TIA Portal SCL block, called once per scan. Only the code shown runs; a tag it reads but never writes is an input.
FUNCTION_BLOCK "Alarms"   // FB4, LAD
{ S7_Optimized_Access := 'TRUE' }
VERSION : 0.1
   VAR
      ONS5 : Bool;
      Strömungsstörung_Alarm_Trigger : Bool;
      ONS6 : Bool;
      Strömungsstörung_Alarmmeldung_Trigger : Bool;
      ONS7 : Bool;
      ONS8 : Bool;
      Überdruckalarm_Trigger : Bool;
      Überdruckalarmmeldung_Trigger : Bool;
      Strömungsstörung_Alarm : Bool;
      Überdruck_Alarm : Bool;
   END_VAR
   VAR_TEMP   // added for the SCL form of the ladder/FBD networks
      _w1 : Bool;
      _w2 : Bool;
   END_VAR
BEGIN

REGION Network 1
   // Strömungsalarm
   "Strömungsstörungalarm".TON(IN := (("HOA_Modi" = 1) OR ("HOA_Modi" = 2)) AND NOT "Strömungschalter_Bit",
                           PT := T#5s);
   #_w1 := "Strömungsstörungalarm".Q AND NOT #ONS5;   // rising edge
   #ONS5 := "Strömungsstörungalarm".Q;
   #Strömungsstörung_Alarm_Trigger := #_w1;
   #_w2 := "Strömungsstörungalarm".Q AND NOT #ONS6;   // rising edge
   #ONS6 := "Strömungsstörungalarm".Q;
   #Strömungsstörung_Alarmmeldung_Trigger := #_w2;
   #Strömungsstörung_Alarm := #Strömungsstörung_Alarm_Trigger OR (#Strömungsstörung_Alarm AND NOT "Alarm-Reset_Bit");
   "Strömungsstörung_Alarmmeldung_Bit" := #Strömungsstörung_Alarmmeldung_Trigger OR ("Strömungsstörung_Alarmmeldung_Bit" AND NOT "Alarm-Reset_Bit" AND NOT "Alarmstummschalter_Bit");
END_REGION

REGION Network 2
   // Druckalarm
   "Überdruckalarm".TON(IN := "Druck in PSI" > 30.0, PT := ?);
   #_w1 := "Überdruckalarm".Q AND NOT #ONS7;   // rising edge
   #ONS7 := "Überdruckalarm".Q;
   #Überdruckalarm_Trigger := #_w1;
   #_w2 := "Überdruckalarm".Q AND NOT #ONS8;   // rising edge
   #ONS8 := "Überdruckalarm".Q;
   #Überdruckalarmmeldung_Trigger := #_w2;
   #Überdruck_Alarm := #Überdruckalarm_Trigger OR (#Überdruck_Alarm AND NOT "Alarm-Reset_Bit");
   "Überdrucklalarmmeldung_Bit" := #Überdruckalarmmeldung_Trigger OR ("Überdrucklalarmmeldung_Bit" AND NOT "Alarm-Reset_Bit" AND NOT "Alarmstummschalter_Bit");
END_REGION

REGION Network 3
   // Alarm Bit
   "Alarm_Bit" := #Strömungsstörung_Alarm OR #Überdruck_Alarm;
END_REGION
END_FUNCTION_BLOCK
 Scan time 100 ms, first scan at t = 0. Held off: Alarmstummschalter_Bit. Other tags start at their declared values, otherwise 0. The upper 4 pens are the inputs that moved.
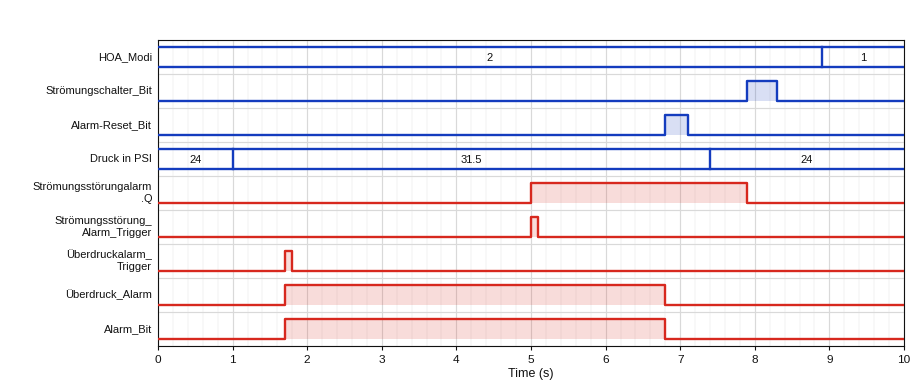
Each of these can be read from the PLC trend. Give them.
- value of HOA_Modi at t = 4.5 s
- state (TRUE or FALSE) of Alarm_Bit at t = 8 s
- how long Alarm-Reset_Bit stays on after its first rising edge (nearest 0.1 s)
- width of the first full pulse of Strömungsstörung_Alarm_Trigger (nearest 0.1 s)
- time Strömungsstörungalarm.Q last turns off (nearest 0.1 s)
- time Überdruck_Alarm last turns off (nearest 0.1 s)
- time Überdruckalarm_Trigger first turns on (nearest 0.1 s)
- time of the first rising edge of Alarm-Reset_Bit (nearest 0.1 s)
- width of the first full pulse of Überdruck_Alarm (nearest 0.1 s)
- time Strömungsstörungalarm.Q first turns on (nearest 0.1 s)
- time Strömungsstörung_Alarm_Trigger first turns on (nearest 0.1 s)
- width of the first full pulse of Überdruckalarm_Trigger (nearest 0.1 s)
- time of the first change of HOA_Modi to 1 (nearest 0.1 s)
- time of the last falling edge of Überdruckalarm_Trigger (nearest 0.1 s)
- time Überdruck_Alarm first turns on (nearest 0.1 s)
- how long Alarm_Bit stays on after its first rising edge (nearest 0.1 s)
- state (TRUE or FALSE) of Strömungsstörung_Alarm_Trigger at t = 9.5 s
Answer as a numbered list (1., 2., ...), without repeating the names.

1. 2
2. FALSE
3. 0.3 s
4. 0.1 s
5. 7.9 s
6. 6.8 s
7. 1.7 s
8. 6.8 s
9. 5.1 s
10. 5.0 s
11. 5.0 s
12. 0.1 s
13. 8.9 s
14. 1.8 s
15. 1.7 s
16. 5.1 s
17. FALSE
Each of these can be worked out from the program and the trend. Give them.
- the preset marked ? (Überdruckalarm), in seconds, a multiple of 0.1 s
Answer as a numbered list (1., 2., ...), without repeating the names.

1. 0.7 s
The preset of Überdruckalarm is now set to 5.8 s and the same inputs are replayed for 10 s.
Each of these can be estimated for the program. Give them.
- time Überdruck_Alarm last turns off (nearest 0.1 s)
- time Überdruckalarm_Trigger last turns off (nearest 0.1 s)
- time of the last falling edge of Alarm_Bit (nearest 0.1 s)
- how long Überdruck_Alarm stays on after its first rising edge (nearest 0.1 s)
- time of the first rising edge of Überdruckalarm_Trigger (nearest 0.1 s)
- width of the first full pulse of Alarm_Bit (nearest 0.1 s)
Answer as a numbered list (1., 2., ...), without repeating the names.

1. 6.9 s
2. 6.9 s
3. 6.9 s
4. 0.1 s
5. 6.8 s
6. 1.9 s
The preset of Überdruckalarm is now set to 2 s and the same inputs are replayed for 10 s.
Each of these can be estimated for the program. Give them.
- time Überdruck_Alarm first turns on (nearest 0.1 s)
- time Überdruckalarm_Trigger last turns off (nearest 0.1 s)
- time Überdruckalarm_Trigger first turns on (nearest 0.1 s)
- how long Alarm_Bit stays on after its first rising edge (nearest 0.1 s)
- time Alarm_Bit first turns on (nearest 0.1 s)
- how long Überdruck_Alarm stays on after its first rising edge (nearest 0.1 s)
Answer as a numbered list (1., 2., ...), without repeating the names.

1. 3.0 s
2. 3.1 s
3. 3.0 s
4. 3.8 s
5. 3.0 s
6. 3.8 s
